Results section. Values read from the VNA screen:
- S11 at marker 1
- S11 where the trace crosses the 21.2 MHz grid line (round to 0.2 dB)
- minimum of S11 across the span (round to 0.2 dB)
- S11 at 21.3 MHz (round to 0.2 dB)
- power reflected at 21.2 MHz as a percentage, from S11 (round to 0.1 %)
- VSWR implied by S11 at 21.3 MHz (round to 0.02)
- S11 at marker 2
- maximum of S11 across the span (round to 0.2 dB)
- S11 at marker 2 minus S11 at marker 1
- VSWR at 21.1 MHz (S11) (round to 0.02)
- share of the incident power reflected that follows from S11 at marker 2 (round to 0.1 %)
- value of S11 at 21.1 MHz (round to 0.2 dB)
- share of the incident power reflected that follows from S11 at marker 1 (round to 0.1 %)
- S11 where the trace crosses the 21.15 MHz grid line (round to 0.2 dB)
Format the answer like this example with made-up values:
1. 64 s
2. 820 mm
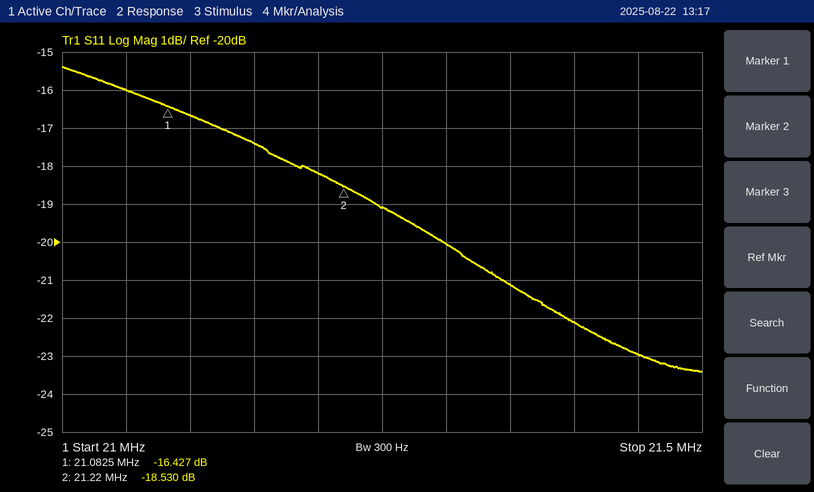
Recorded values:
1. -16.427 dB
2. -18.2 dB
3. -23.4 dB
4. -20.0 dB
5. 1.5 %
6. 1.22
7. -18.530 dB
8. -15.4 dB
9. -2.103 dB
10. 1.34
11. 1.4 %
12. -16.6 dB
13. 2.3 %
14. -17.4 dB
